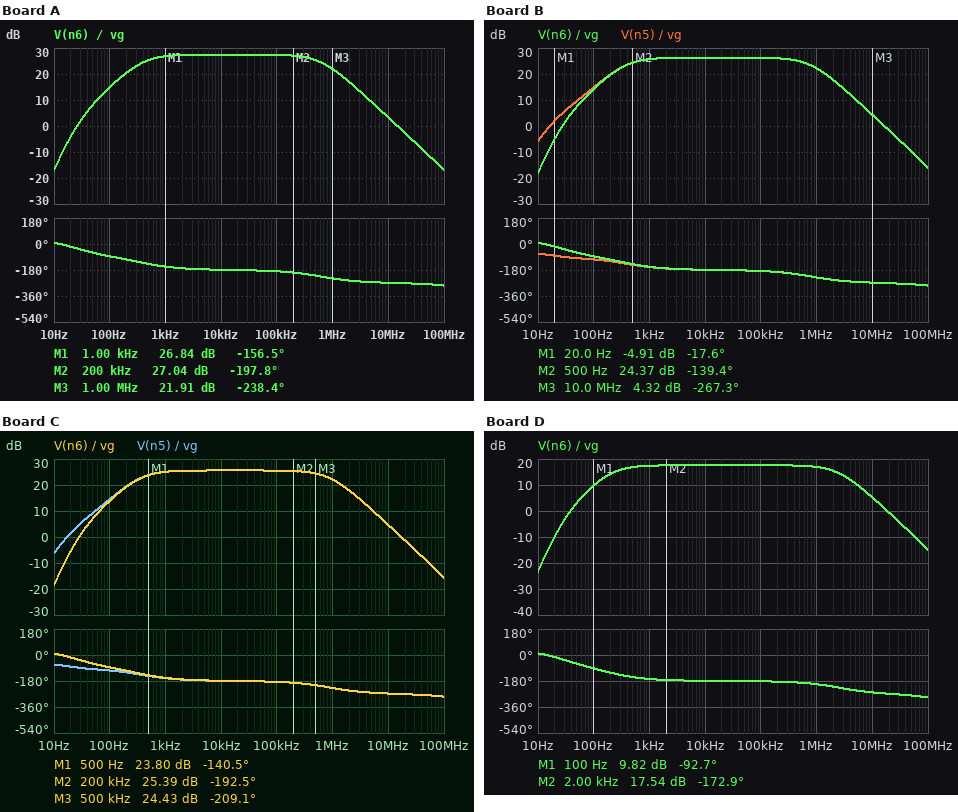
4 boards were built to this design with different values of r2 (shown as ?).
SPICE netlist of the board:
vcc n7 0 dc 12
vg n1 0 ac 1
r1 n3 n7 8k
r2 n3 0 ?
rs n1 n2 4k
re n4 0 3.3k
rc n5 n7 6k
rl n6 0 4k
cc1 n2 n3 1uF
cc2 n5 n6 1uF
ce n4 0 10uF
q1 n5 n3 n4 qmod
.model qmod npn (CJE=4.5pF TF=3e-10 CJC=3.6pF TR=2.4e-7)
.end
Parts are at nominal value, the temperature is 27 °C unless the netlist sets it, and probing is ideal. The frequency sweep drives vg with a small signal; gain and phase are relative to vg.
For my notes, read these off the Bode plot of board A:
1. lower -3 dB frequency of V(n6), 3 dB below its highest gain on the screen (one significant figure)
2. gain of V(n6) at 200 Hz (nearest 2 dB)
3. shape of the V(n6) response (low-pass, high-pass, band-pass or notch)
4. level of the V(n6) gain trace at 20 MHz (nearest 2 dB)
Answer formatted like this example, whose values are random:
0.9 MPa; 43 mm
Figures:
400 Hz; 20 dB; band-pass; -2 dB
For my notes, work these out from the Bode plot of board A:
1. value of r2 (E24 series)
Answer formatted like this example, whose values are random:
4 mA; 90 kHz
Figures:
4.3 kΩ
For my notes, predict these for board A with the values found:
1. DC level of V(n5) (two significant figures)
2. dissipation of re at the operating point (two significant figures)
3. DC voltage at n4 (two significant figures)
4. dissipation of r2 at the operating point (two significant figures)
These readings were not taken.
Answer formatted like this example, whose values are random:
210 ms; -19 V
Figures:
5.9 V; 3.5 mW; 3.4 V; 4.0 mW
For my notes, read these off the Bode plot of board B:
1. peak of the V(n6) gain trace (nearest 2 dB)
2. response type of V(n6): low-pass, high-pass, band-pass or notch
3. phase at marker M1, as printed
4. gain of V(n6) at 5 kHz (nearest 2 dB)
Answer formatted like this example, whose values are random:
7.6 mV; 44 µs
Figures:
26 dB; band-pass; -17.6 deg; 26 dB
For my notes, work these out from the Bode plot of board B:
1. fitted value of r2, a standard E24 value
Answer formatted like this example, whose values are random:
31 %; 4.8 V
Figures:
3.6 kΩ
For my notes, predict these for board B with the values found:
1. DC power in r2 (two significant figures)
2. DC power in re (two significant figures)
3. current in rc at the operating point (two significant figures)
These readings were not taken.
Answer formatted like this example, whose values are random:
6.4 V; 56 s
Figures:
3.8 mW; 2.6 mW; 880 µA
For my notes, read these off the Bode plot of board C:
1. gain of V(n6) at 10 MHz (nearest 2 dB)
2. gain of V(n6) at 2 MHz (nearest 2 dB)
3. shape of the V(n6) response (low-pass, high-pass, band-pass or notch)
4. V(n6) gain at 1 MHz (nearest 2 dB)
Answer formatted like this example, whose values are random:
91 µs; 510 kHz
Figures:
4 dB; 18 dB; band-pass; 22 dB
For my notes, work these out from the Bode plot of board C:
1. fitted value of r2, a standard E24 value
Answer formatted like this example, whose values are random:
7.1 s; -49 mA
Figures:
3.3 kΩ
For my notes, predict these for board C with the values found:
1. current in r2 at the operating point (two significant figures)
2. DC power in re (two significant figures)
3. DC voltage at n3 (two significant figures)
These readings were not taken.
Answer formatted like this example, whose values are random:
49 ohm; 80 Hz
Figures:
1.1 mA; 2.2 mW; 3.5 V
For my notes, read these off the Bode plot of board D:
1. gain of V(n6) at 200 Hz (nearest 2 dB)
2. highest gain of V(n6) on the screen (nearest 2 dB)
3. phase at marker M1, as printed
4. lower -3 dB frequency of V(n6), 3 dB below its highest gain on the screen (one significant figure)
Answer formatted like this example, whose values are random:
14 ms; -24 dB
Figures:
14 dB; 18 dB; -92.7 deg; 200 Hz
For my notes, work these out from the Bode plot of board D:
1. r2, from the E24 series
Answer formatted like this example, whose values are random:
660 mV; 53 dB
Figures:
1.6 kΩ
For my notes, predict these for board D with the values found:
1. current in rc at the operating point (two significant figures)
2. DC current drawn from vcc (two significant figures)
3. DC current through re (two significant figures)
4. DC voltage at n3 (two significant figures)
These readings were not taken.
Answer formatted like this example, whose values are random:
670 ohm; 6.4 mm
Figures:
370 µA; 1.6 mA; 380 µA; 2.0 V
